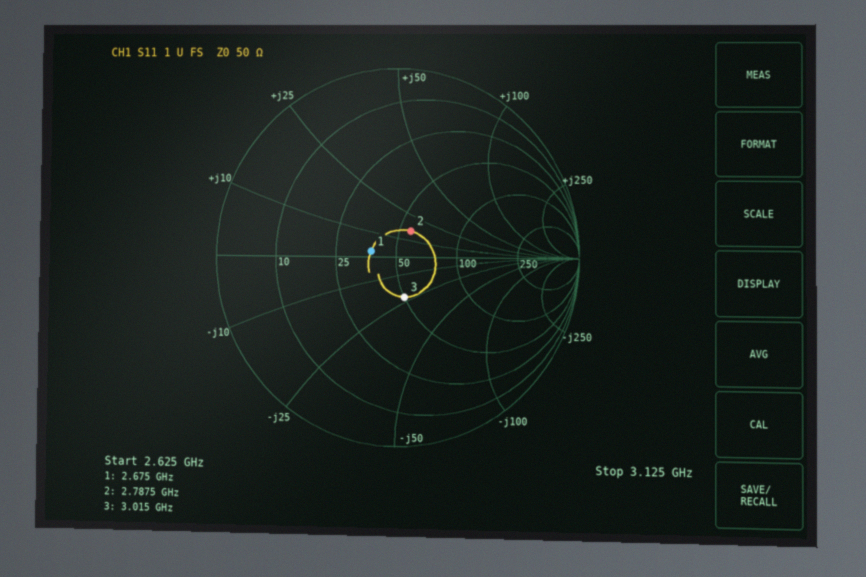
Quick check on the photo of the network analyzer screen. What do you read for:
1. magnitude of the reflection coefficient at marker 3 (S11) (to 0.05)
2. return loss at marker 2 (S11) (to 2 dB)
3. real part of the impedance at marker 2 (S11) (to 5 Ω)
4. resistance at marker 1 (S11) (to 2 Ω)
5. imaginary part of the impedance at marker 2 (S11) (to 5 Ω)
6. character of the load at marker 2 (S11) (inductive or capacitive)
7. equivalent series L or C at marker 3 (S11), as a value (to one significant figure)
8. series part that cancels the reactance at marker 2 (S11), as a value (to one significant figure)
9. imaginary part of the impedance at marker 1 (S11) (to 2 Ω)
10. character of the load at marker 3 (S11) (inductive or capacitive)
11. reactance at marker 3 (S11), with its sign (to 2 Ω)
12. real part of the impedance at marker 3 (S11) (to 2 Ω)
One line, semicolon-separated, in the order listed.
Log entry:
0.20; 16 dB; 55 Ω; 38 Ω; +15 Ω; inductive; 2 pF; 4 pF; +2 Ω; capacitive; -22 Ω; 50 Ω
